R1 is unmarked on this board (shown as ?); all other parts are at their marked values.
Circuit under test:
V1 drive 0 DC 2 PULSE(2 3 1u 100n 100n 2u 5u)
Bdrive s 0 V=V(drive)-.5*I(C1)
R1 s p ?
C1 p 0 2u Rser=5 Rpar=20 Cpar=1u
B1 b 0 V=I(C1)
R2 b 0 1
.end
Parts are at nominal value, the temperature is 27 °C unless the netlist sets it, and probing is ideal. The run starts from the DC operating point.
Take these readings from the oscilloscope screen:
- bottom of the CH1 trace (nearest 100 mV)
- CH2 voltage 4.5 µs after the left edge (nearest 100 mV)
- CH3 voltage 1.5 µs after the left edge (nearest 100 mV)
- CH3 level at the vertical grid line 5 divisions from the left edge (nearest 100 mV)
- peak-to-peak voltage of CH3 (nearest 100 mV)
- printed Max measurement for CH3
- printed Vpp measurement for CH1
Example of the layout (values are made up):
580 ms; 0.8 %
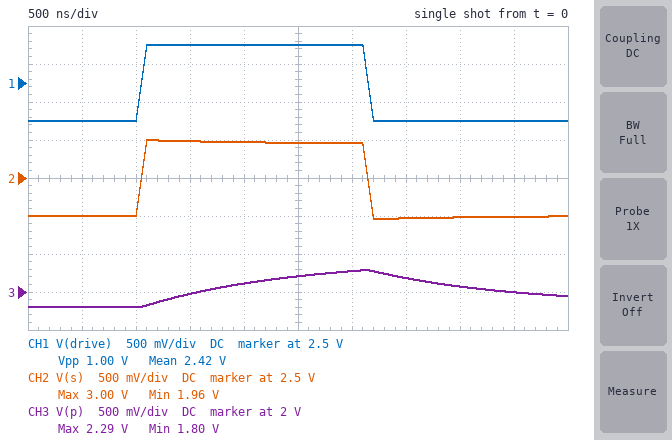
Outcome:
2.0 V; 2.0 V; 2.0 V; 2.2 V; 500 mV; 2.29 V; 1.00 V
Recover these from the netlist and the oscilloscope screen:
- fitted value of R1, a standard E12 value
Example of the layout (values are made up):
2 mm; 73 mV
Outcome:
2.2 Ω
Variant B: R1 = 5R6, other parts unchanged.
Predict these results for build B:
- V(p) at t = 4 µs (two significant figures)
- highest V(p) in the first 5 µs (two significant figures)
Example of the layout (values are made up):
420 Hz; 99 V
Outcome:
1.7 V; 1.8 V
